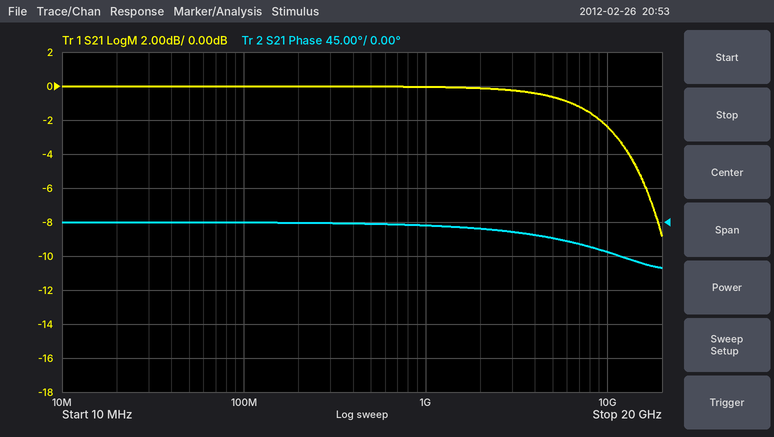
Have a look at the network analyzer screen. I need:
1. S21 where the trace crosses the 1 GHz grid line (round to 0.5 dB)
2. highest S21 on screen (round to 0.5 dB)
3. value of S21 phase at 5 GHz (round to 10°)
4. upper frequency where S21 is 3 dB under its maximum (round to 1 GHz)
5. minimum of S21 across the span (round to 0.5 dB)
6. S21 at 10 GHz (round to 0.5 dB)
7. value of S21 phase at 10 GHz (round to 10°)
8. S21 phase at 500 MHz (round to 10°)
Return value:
0.0 dB
0.0 dB
-20°
11 GHz
-9.0 dB
-2.5 dB
-40°
0°
